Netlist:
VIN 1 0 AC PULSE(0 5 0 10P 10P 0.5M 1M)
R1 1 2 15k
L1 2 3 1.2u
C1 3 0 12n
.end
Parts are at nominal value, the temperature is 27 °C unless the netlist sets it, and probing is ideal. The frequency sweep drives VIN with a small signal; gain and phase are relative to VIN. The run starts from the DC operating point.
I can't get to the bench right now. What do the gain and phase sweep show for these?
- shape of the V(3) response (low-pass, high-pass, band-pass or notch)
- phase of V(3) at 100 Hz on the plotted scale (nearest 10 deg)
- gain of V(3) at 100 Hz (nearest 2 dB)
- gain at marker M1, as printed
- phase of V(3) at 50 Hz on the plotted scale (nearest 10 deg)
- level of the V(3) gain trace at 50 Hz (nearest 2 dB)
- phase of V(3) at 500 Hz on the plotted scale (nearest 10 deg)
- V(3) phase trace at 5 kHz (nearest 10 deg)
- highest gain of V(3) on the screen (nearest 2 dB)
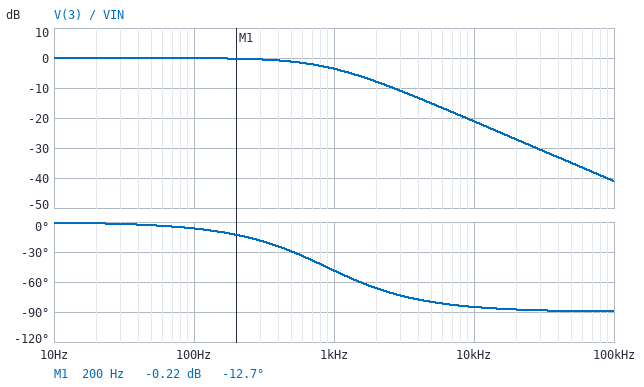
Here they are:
low-pass
-10 deg
0 dB
-0.22 dB
0 deg
0 dB
-30 deg
-80 deg
0 dB
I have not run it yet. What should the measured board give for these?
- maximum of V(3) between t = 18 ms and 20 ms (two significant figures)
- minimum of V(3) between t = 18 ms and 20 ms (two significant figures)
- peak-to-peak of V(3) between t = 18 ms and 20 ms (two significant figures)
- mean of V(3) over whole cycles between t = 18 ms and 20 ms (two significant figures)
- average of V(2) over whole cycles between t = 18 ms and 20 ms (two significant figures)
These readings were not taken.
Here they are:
4.7 V
290 mV
4.4 V
2.5 V
2.5 V
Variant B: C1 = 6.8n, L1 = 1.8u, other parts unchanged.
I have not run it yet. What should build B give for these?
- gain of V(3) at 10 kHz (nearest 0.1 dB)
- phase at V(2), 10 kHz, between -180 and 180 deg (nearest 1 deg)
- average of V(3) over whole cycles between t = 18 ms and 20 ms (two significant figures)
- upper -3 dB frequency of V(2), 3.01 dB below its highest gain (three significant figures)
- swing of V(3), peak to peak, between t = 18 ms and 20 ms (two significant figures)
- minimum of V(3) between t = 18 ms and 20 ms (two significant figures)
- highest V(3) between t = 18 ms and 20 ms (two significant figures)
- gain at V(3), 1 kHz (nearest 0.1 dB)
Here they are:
-16.2 dB
-81 deg
2.5 V
1.56 kHz
4.9 V
37 mV
5.0 V
-1.5 dB
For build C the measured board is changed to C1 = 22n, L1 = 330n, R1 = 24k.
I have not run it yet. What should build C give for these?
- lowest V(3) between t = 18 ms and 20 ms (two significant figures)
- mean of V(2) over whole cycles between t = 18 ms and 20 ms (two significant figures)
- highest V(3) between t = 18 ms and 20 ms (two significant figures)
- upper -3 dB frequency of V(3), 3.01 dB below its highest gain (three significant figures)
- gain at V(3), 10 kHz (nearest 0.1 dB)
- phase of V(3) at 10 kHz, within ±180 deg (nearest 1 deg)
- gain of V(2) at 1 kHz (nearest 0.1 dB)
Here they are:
1.4 V
2.5 V
3.6 V
301 Hz
-30.4 dB
-88 deg
-10.8 dB
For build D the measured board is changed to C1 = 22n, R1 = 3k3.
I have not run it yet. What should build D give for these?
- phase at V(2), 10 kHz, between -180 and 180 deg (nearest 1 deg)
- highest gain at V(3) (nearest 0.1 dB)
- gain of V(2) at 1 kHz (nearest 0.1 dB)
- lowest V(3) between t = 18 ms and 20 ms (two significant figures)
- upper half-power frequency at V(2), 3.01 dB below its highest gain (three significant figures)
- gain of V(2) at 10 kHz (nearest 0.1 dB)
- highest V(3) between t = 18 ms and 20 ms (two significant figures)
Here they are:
-78 deg
0 dB
-0.8 dB
5.1 mV
2.19 kHz
-13.4 dB
5.0 V
